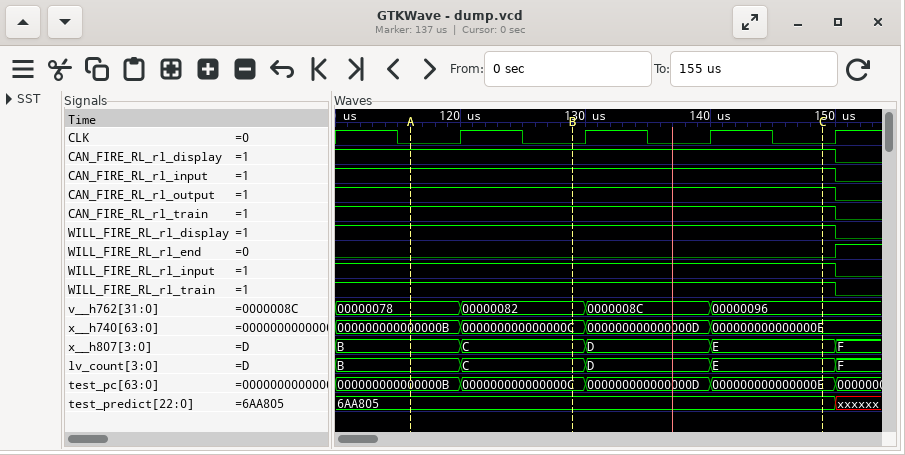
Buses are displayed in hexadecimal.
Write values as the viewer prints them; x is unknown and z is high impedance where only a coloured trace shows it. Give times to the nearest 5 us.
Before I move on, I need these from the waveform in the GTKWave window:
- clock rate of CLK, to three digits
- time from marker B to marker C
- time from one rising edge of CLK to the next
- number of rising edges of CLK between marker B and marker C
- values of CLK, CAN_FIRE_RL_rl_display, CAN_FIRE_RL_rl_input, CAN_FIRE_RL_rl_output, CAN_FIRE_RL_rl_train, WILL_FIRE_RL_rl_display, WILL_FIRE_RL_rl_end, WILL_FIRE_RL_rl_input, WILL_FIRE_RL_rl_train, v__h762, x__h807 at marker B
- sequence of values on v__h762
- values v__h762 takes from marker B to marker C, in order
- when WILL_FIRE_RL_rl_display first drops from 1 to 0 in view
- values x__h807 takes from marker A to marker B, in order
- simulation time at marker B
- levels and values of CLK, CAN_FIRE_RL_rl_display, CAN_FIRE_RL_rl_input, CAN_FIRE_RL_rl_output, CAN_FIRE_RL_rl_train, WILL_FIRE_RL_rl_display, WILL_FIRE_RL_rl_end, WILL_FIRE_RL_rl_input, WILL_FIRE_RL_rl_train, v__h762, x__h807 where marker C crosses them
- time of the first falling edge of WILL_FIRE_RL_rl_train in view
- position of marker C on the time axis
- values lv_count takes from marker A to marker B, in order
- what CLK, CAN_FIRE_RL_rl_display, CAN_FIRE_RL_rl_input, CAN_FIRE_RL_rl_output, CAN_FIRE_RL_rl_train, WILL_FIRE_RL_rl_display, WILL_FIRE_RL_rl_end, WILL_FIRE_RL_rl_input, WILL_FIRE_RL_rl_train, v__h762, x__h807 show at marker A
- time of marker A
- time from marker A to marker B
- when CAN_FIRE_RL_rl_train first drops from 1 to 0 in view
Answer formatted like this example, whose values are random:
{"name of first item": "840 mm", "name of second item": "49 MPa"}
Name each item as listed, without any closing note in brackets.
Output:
{"clock rate of CLK, to three digits": "100 kHz", "time from marker B to marker C": "20 us", "time from one rising edge of CLK to the next": "10 us", "number of rising edges of CLK between marker B and marker C": "2", "values of CLK, CAN_FIRE_RL_rl_display, CAN_FIRE_RL_rl_input, CAN_FIRE_RL_rl_output, CAN_FIRE_RL_rl_train, WILL_FIRE_RL_rl_display, WILL_FIRE_RL_rl_end, WILL_FIRE_RL_rl_input, WILL_FIRE_RL_rl_train, v__h762, x__h807 at marker B": "CLK=0, CAN_FIRE_RL_rl_display=1, CAN_FIRE_RL_rl_input=1, CAN_FIRE_RL_rl_output=1, CAN_FIRE_RL_rl_train=1, WILL_FIRE_RL_rl_display=1, WILL_FIRE_RL_rl_end=0, WILL_FIRE_RL_rl_input=1, WILL_FIRE_RL_rl_train=1, v__h762=00000082, x__h807=C", "sequence of values on v__h762": "00000078, 00000082, 0000008C, 00000096", "values v__h762 takes from marker B to marker C, in order": "00000082, 0000008C, 00000096", "when WILL_FIRE_RL_rl_display first drops from 1 to 0 in view": "150 us", "values x__h807 takes from marker A to marker B, in order": "B, C", "simulation time at marker B": "130 us", "levels and values of CLK, CAN_FIRE_RL_rl_display, CAN_FIRE_RL_rl_input, CAN_FIRE_RL_rl_output, CAN_FIRE_RL_rl_train, WILL_FIRE_RL_rl_display, WILL_FIRE_RL_rl_end, WILL_FIRE_RL_rl_input, WILL_FIRE_RL_rl_train, v__h762, x__h807 where marker C crosses them": "CLK=0, CAN_FIRE_RL_rl_display=1, CAN_FIRE_RL_rl_input=1, CAN_FIRE_RL_rl_output=1, CAN_FIRE_RL_rl_train=1, WILL_FIRE_RL_rl_display=1, WILL_FIRE_RL_rl_end=0, WILL_FIRE_RL_rl_input=1, WILL_FIRE_RL_rl_train=1, v__h762=00000096, x__h807=E", "time of the first falling edge of WILL_FIRE_RL_rl_train in view": "150 us", "position of marker C on the time axis": "150 us", "values lv_count takes from marker A to marker B, in order": "B, C", "what CLK, CAN_FIRE_RL_rl_display, CAN_FIRE_RL_rl_input, CAN_FIRE_RL_rl_output, CAN_FIRE_RL_rl_train, WILL_FIRE_RL_rl_display, WILL_FIRE_RL_rl_end, WILL_FIRE_RL_rl_input, WILL_FIRE_RL_rl_train, v__h762, x__h807 show at marker A": "CLK=0, CAN_FIRE_RL_rl_display=1, CAN_FIRE_RL_rl_input=1, CAN_FIRE_RL_rl_output=1, CAN_FIRE_RL_rl_train=1, WILL_FIRE_RL_rl_display=1, WILL_FIRE_RL_rl_end=0, WILL_FIRE_RL_rl_input=1, WILL_FIRE_RL_rl_train=1, v__h762=00000078, x__h807=B", "time of marker A": "115 us", "time from marker A to marker B": "15 us", "when CAN_FIRE_RL_rl_train first drops from 1 to 0 in view": "150 us"}
